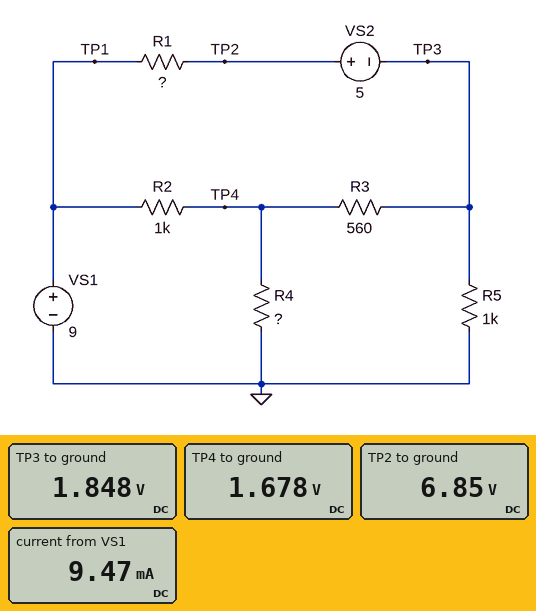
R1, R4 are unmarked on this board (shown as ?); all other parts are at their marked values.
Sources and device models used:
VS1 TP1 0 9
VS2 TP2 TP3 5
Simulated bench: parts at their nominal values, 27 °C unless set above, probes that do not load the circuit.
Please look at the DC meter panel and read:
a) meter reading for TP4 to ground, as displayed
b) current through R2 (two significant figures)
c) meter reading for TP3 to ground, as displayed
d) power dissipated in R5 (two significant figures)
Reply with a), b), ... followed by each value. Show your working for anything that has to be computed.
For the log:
a) 1.678 V
b) (9 V - 1.678 V) / 1 kΩ = 7.3 mA
c) 1.848 V
d) (1.848 V)^2 / 1 kΩ = 3.4 mW
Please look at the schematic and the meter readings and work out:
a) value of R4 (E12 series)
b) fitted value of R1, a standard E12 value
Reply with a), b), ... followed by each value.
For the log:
a) 220 Ω
b) 1 kΩ
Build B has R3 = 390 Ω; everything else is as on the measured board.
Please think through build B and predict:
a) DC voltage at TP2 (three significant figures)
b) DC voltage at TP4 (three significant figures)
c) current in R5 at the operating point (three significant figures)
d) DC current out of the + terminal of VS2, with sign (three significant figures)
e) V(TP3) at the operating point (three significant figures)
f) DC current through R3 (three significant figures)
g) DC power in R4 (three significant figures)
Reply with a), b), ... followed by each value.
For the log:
a) 6.82 V
b) 1.69 V
c) 1.82 mA
d) -2.18 mA
e) 1.82 V
f) 352 µA
g) 12.9 mW
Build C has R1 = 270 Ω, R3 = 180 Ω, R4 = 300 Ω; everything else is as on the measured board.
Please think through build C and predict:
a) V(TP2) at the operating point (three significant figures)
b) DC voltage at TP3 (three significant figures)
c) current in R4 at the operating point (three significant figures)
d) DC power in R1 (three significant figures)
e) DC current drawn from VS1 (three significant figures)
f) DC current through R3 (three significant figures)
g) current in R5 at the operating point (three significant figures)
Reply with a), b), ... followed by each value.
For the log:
a) 7.78 V
b) 2.78 V
c) 8.25 mA
d) 5.48 mW
e) 11.0 mA
f) 1.72 mA
g) 2.78 mA
